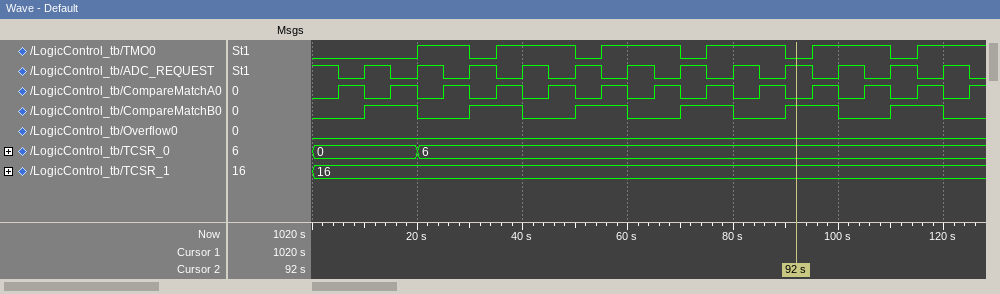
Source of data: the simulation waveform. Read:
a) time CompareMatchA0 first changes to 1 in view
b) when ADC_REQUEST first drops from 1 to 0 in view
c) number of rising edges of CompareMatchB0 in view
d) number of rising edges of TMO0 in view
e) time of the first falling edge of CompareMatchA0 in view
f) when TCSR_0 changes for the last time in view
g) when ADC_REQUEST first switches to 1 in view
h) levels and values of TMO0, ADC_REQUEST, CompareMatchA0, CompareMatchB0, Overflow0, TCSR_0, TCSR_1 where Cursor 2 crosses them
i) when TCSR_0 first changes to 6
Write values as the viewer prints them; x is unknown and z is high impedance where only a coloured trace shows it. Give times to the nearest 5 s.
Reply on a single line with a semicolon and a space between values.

5 s; 5 s; 6; 6; 10 s; 20 s; 10 s; TMO0=0, ADC_REQUEST=1, CompareMatchA0=0, CompareMatchB0=1, Overflow0=0, TCSR_0=6, TCSR_1=16; 20 s
